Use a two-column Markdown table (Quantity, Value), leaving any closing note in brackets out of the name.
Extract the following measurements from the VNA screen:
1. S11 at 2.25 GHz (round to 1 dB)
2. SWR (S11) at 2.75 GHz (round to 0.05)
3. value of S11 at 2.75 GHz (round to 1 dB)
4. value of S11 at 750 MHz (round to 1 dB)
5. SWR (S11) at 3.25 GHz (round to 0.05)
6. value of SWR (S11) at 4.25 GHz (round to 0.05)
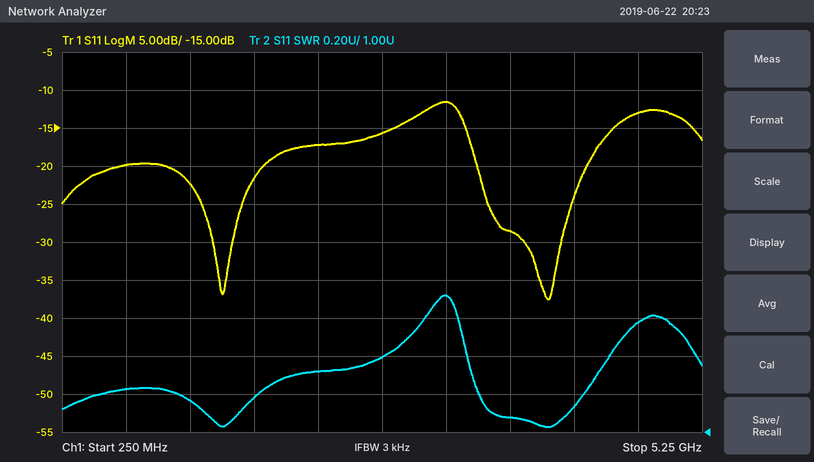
| Quantity | Value |
|---|---|
| S11 at 2.25 GHz | -17 dB |
| SWR (S11) at 2.75 GHz | 1.40 |
| value of S11 at 2.75 GHz | -16 dB |
| value of S11 at 750 MHz | -20 dB |
| SWR (S11) at 3.25 GHz | 1.70 |
| value of SWR (S11) at 4.25 GHz | 1.15 |
